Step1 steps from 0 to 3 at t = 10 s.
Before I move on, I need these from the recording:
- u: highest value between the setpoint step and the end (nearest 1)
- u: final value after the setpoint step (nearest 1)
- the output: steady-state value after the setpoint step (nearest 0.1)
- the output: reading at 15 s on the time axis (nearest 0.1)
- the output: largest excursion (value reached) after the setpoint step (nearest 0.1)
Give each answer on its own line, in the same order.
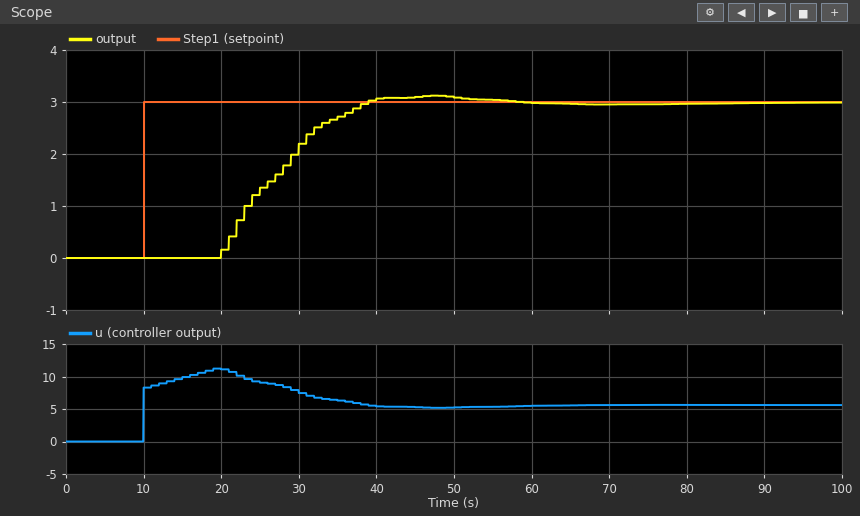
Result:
11
6
3.0
0.0
3.1
